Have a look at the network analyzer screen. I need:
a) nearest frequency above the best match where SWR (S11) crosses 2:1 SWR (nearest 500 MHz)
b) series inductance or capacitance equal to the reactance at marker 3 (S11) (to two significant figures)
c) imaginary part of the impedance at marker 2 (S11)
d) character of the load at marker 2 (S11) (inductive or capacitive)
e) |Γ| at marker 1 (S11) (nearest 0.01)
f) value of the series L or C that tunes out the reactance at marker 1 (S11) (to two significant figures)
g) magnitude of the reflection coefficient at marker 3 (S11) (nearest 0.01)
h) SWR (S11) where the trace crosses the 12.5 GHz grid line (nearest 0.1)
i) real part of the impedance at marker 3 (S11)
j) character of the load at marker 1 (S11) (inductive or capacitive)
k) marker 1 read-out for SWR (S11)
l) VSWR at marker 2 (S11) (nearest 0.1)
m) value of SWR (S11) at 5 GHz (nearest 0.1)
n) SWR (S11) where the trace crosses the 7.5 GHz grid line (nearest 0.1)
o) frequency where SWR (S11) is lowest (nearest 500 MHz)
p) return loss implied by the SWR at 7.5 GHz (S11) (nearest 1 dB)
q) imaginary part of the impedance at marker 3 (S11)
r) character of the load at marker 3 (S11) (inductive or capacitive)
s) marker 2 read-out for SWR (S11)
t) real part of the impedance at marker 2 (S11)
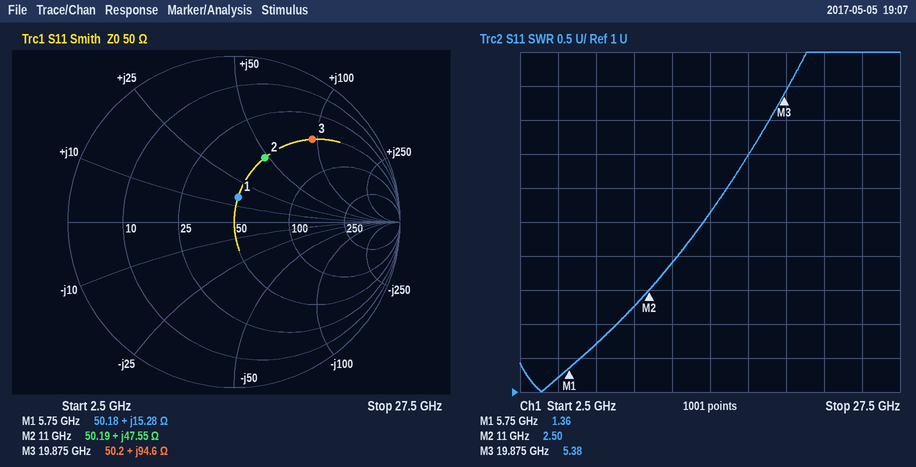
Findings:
9.0 GHz
760 pH
+47.55 Ω
inductive
0.15
1.8 pF
0.69
2.9
50.2 Ω
inductive
1.36
2.5
1.2
1.7
4.0 GHz
12 dB
+94.6 Ω
inductive
2.50
50.19 Ω
